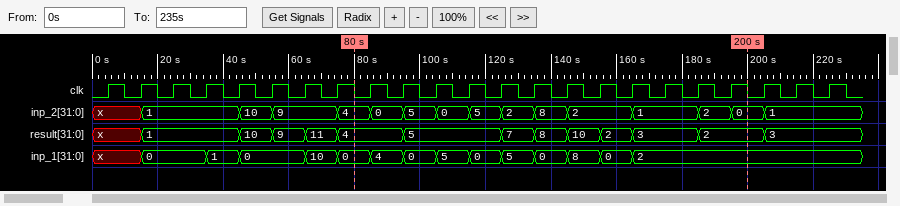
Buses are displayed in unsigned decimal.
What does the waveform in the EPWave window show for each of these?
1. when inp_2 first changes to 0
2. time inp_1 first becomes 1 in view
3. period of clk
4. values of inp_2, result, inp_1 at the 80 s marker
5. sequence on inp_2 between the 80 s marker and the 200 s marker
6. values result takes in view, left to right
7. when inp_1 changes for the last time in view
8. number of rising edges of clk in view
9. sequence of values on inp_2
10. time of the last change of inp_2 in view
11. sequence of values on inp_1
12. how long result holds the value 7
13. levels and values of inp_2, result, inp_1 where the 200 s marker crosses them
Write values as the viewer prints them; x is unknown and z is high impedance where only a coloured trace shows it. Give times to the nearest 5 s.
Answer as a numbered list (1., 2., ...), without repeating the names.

1. 85 s
2. 35 s
3. 10 s
4. inp_2=4, result=4, inp_1=0
5. 4, 0, 5, 0, 5, 2, 8, 2, 1, 2, 0
6. x, 1, 10, 9, 11, 4, 5, 7, 8, 10, 2, 3, 2, 3
7. 165 s
8. 23
9. x, 1, 10, 9, 4, 0, 5, 0, 5, 2, 8, 2, 1, 2, 0, 1
10. 205 s
11. x, 0, 1, 0, 10, 0, 4, 0, 5, 0, 5, 0, 8, 0, 2
12. 10 s
13. inp_2=0, result=2, inp_1=2
